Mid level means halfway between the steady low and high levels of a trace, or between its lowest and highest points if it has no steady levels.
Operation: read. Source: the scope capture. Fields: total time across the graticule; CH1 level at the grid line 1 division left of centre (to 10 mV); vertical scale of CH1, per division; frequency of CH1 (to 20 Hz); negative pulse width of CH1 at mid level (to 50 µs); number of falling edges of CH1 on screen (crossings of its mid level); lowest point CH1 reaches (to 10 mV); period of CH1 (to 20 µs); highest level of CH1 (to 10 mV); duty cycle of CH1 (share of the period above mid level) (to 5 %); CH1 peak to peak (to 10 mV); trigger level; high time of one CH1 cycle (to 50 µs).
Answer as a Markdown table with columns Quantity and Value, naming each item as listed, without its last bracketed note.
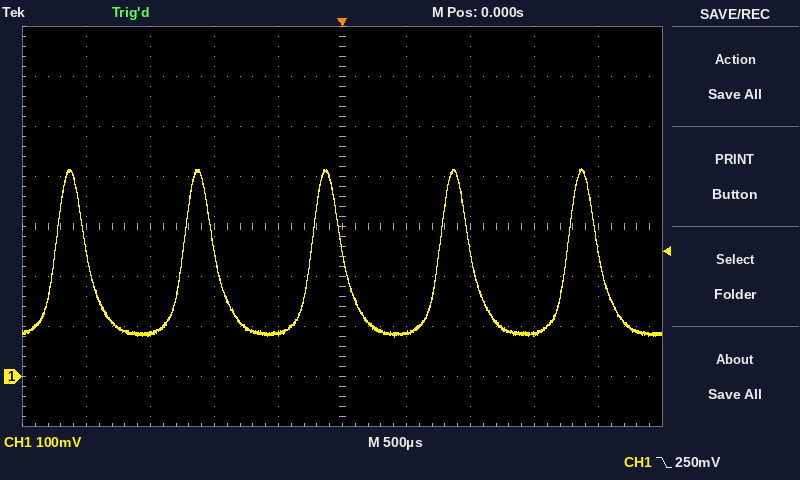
| Quantity | Value |
|---|---|
| total time across the graticule | 5 ms |
| CH1 level at the grid line 1 division left of centre | 90 mV |
| vertical scale of CH1, per division | 100 mV |
| frequency of CH1 | 1.00 kHz |
| negative pulse width of CH1 at mid level | 750 µs |
| number of falling edges of CH1 on screen | 5 |
| lowest point CH1 reaches | 80 mV |
| period of CH1 | 1.00 ms |
| highest level of CH1 | 420 mV |
| duty cycle of CH1 (share of the period above mid level) | 25 % |
| CH1 peak to peak | 340 mV |
| trigger level | 250 mV |
| high time of one CH1 cycle | 250 µs |
